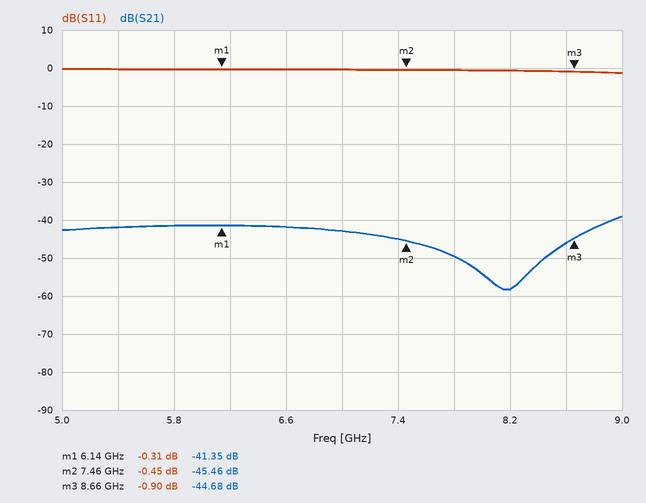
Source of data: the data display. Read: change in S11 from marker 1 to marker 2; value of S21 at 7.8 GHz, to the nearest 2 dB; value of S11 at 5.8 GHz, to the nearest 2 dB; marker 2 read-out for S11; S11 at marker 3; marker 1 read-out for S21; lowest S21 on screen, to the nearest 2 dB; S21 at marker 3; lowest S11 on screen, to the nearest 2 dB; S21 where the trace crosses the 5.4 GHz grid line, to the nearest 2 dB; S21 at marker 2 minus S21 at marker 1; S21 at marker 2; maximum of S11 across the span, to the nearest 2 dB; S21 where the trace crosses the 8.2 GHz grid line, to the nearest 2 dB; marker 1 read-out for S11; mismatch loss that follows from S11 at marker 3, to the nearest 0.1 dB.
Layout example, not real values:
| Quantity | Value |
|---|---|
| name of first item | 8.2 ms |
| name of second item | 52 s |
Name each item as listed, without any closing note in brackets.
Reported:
| Quantity | Value |
|---|---|
| change in S11 from marker 1 to marker 2 | -0.14 dB |
| value of S21 at 7.8 GHz, to the nearest 2 dB | -50 dB |
| value of S11 at 5.8 GHz, to the nearest 2 dB | 0 dB |
| marker 2 read-out for S11 | -0.45 dB |
| S11 at marker 3 | -0.90 dB |
| marker 1 read-out for S21 | -41.35 dB |
| lowest S21 on screen, to the nearest 2 dB | -58 dB |
| S21 at marker 3 | -44.68 dB |
| lowest S11 on screen, to the nearest 2 dB | -2 dB |
| S21 where the trace crosses the 5.4 GHz grid line, to the nearest 2 dB | -42 dB |
| S21 at marker 2 minus S21 at marker 1 | -4.11 dB |
| S21 at marker 2 | -45.46 dB |
| maximum of S11 across the span, to the nearest 2 dB | 0 dB |
| S21 where the trace crosses the 8.2 GHz grid line, to the nearest 2 dB | -58 dB |
| marker 1 read-out for S11 | -0.31 dB |
| mismatch loss that follows from S11 at marker 3, to the nearest 0.1 dB | 7.3 dB |
